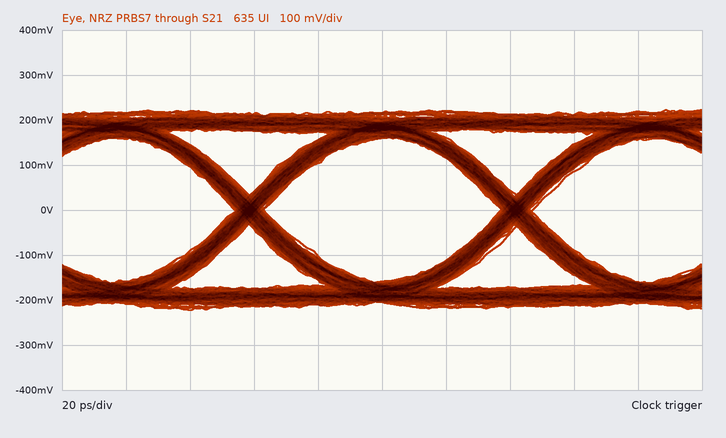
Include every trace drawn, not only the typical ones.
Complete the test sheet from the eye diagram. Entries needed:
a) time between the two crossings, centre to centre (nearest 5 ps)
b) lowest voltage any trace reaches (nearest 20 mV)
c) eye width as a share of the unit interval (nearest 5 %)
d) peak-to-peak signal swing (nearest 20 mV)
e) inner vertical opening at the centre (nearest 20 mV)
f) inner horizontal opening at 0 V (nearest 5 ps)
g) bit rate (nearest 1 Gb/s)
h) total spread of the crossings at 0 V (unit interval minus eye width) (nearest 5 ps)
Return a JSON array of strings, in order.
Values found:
["85 ps", "-220 mV", "90 %", "440 mV", "320 mV", "75 ps", "12 Gb/s", "10 ps"]
